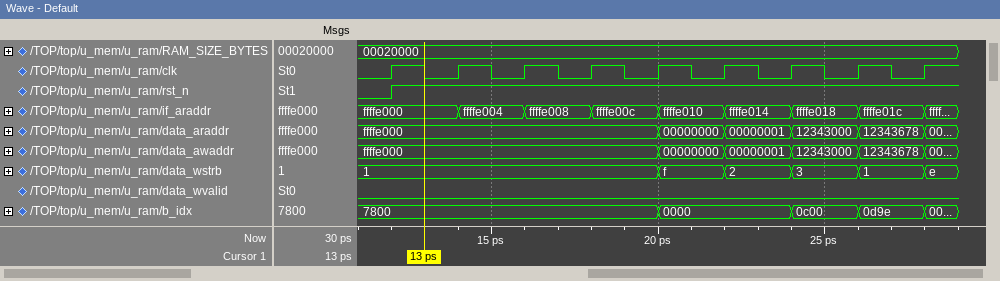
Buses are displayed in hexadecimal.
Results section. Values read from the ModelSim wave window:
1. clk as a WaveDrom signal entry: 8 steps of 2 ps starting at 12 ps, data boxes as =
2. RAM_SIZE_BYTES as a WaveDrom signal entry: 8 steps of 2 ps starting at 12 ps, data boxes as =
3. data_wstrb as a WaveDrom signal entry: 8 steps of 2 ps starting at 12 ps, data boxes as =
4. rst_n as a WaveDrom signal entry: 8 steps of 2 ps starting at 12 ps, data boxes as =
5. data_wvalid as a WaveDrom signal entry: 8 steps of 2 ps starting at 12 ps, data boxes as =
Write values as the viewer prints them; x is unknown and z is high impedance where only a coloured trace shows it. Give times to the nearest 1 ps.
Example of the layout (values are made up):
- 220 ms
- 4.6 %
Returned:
- {name: 'clk', wave: 'p.......'}
- {name: 'RAM_SIZE_BYTES', wave: '=.......', data: '00020000'}
- {name: 'data_wstrb', wave: '=...====', data: '1 f 2 3 1'}
- {name: 'rst_n', wave: '1.......'}
- {name: 'data_wvalid', wave: '0.......'}
